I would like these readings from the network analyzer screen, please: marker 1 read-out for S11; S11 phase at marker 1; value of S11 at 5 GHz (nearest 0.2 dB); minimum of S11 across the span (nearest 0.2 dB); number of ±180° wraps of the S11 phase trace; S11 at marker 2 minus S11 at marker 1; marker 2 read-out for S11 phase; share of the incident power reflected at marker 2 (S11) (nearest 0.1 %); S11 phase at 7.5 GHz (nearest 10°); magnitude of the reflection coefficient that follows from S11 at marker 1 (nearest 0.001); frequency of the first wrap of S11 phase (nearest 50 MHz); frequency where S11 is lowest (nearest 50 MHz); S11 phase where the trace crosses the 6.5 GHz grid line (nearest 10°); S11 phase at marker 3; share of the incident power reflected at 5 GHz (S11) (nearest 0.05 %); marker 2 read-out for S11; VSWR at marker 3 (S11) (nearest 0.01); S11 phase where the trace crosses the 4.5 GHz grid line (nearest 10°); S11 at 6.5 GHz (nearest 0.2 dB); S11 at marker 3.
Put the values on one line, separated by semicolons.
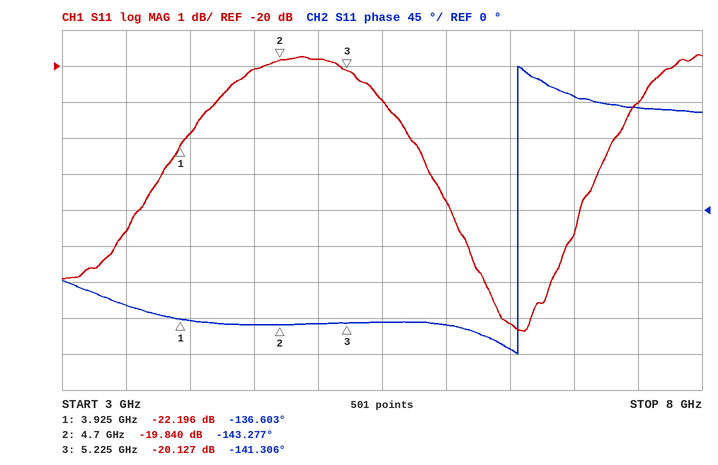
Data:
-22.196 dB; -136.603°; -19.8 dB; -27.4 dB; 1; 2.356 dB; -143.277°; 1.0 %; 130°; 0.078; 6.55 GHz; 6.60 GHz; -170°; -141.306°; 1.05 %; -19.840 dB; 1.22; -140°; -27.2 dB; -20.127 dB
